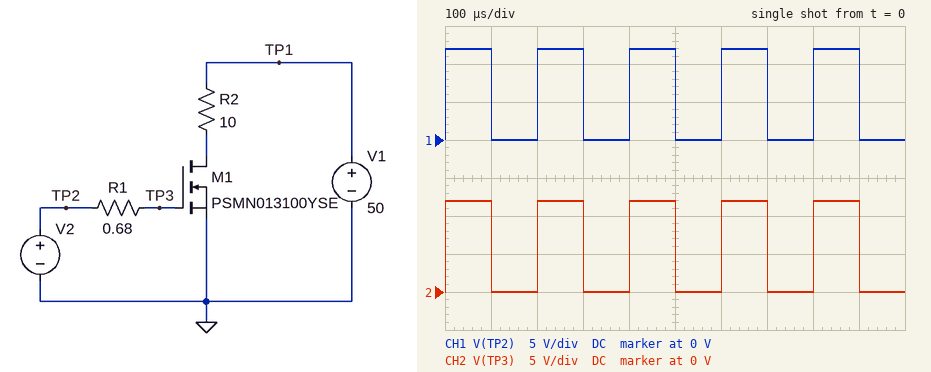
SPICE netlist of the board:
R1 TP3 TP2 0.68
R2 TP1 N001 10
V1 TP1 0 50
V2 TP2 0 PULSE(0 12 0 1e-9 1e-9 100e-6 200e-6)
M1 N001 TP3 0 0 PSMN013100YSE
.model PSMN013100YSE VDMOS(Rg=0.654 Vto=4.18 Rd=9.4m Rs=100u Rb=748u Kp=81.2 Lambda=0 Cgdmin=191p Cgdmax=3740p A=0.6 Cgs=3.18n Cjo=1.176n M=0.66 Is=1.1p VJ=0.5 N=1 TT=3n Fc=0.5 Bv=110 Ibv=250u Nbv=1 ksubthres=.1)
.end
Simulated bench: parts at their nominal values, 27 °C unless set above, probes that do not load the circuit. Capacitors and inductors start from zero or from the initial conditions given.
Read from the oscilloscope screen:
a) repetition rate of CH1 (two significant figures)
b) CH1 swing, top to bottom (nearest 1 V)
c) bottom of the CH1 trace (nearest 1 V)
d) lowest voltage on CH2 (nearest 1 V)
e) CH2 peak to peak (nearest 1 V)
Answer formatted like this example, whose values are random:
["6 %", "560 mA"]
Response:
["5.0 kHz", "12 V", "0 V", "0 V", "12 V"]
